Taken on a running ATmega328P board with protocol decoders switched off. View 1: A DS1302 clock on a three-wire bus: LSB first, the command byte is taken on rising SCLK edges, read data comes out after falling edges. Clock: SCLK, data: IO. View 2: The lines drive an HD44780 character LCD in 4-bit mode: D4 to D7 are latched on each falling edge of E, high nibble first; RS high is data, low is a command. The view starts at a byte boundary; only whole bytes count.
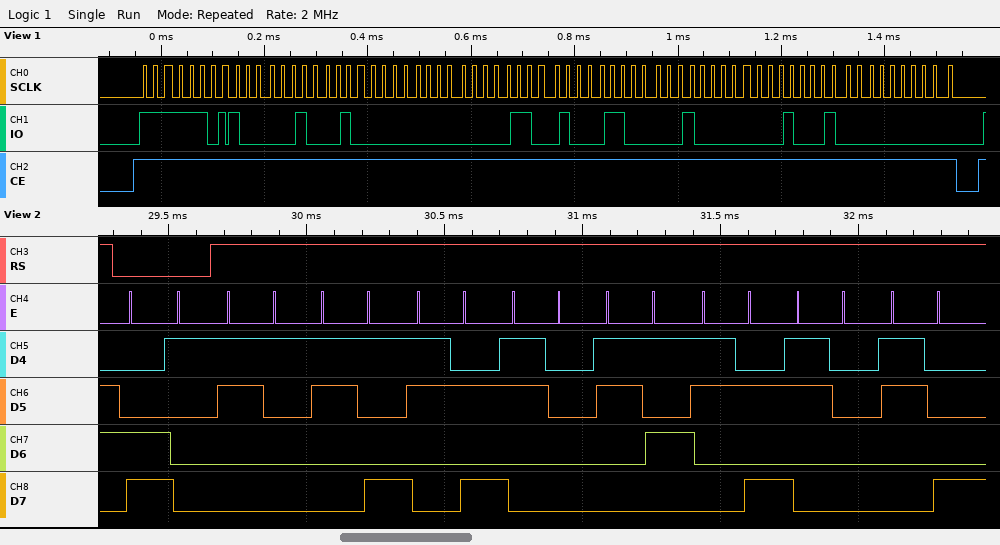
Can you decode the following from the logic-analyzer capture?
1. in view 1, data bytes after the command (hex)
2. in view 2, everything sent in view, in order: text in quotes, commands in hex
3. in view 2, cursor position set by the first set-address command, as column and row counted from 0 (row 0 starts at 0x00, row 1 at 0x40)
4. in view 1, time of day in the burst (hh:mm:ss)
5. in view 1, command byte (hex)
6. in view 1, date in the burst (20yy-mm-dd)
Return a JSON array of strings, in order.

["41 04 00 26 06 01 22 00", "0xC1 \"19:05:08\"", "column 1, row 1", "00:04:41", "0xBF", "2022-06-26"]
